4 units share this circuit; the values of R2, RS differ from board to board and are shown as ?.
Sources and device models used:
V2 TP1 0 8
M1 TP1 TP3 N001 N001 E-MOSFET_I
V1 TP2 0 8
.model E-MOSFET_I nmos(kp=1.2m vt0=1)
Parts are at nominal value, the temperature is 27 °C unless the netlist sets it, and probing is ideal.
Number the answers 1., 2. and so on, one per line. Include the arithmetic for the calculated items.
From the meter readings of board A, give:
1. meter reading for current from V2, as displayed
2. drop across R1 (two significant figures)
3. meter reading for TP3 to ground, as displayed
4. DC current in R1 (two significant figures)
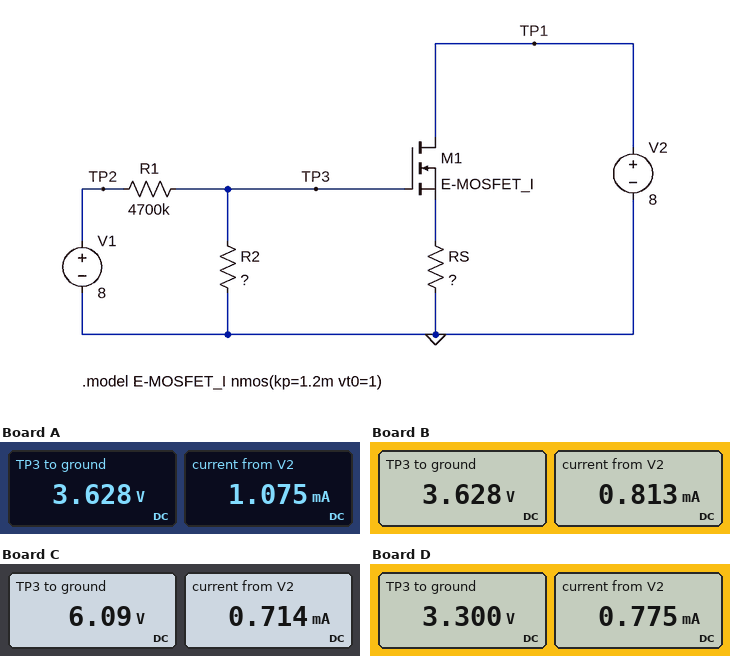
1. 1.075 mA
2. 8 V - 3.628 V = 4.4 V
3. 3.628 V
4. (8 V - 3.628 V) / 4.7 MΩ = 930 nA
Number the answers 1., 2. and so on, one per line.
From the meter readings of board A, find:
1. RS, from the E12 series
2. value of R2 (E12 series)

1. 1.2 kΩ
2. 3.9 MΩ
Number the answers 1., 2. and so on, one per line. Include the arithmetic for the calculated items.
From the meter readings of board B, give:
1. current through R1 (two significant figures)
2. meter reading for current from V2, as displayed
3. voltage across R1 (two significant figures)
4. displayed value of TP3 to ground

1. (8 V - 3.628 V) / 4.7 MΩ = 930 nA
2. 0.813 mA
3. 8 V - 3.628 V = 4.4 V
4. 3.628 V
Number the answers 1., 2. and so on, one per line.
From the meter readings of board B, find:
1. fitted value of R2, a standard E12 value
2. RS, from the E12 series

1. 3.9 MΩ
2. 1.8 kΩ
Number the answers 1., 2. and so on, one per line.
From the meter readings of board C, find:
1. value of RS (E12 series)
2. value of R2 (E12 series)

1. 5.6 kΩ
2. 15 MΩ
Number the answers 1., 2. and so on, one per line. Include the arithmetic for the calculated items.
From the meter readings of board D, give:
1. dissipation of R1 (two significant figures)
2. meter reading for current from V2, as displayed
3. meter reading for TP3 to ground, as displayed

1. (8 V - 3.3 V)^2 / 4.7 MΩ = 4.7 µW
2. 0.775 mA
3. 3.300 V
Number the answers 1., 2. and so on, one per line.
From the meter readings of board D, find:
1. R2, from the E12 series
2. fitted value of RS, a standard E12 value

1. 3.3 MΩ
2. 1.5 kΩ
